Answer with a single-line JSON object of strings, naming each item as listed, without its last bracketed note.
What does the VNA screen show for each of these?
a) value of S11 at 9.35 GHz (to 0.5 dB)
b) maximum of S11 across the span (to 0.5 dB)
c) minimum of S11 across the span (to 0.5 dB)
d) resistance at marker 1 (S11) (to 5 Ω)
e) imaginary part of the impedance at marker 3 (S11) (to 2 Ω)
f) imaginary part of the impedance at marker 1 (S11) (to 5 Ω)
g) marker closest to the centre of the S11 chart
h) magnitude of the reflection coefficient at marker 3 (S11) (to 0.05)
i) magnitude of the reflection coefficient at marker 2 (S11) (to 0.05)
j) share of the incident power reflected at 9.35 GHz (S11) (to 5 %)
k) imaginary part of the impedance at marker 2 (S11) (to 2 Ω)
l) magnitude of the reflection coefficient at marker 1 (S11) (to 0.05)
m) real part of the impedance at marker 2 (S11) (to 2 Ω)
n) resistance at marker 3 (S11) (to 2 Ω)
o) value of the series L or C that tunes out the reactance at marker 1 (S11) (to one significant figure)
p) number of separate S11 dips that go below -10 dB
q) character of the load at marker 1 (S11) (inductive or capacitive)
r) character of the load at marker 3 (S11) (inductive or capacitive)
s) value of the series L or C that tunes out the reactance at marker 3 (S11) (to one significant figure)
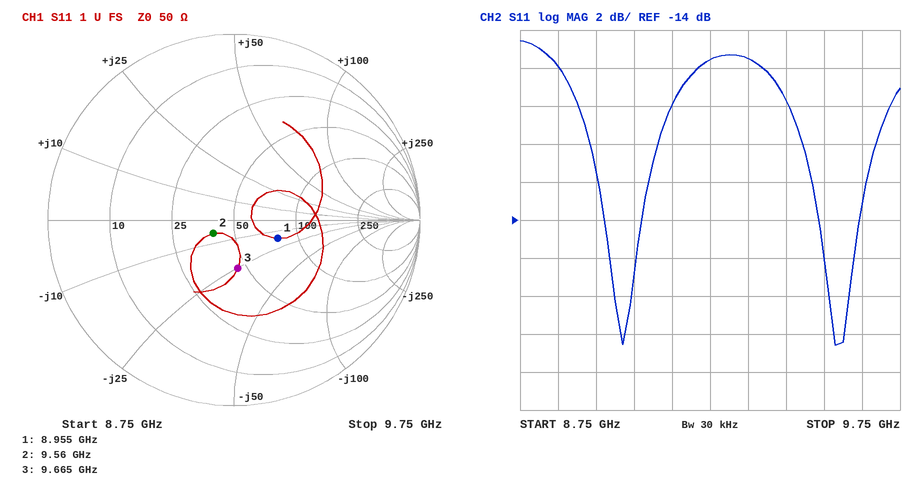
{"value of S11 at 9.35 GHz": "-5.5 dB", "maximum of S11 across the span": "-4.5 dB", "minimum of S11 across the span": "-20.5 dB", "resistance at marker 1 (S11)": "80 Ω", "imaginary part of the impedance at marker 3 (S11)": "-26 Ω", "imaginary part of the impedance at marker 1 (S11)": "-15 Ω", "marker closest to the centre of the S11 chart": "marker 2", "magnitude of the reflection coefficient at marker 3 (S11)": "0.25", "magnitude of the reflection coefficient at marker 2 (S11)": "0.15", "share of the incident power reflected at 9.35 GHz (S11)": "30 %", "imaginary part of the impedance at marker 2 (S11)": "-6 Ω", "magnitude of the reflection coefficient at marker 1 (S11)": "0.25", "real part of the impedance at marker 2 (S11)": "40 Ω", "resistance at marker 3 (S11)": "46 Ω", "value of the series L or C that tunes out the reactance at marker 1 (S11)": "300 pH", "number of separate S11 dips that go below -10 dB": "2", "character of the load at marker 1 (S11)": "capacitive", "character of the load at marker 3 (S11)": "capacitive", "value of the series L or C that tunes out the reactance at marker 3 (S11)": "400 pH"}
